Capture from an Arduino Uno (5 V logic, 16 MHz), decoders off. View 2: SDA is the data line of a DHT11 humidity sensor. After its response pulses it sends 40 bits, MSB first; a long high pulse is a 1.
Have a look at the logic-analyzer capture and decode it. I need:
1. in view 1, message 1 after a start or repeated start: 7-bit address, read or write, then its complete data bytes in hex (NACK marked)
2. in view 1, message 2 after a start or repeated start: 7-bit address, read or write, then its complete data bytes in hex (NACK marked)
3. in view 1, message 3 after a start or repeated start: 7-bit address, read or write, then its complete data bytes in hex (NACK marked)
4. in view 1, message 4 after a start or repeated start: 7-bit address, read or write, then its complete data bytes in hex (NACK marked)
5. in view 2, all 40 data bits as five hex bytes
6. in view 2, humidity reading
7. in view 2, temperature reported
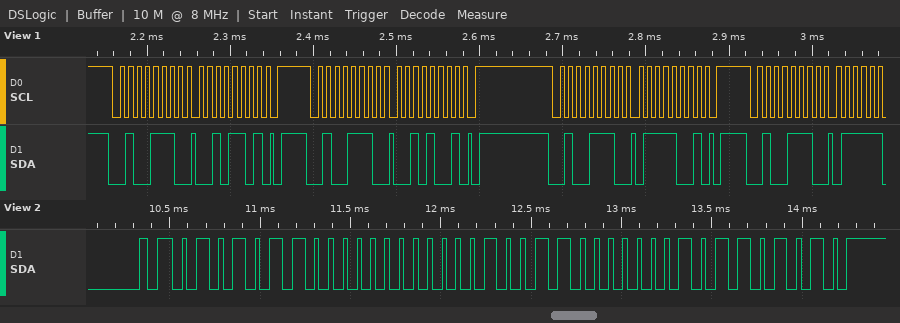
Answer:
0x27 write: 2D
0x27 write: 29
0x27 write: 79
0x27 write
56 00 13 01 6A
86 %
19.1 °C
